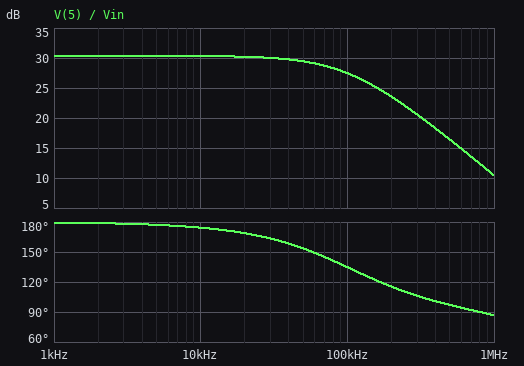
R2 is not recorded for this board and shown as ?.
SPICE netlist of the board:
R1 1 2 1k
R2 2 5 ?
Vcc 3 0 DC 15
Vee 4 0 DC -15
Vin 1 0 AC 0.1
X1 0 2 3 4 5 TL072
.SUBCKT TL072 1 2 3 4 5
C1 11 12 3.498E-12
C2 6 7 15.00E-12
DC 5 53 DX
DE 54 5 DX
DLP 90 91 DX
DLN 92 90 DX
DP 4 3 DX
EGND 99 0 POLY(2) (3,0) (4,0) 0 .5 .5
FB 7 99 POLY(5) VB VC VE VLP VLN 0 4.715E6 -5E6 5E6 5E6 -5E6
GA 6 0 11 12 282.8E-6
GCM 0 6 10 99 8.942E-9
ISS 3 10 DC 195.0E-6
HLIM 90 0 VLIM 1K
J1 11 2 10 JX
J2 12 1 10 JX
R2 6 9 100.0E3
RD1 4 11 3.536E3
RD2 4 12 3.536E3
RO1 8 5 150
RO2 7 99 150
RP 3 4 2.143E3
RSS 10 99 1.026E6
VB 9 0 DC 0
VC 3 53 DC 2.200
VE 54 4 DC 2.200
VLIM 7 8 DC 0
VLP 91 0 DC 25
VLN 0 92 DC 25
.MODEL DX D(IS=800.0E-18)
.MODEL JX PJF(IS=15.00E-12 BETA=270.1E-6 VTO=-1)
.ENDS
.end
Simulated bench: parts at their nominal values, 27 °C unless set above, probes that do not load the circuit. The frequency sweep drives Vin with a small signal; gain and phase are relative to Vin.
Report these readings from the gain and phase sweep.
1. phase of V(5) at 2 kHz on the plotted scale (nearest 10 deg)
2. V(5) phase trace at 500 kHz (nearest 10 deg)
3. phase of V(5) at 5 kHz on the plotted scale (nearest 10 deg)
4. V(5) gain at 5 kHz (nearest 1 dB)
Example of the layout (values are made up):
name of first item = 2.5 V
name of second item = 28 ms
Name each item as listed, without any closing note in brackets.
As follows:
phase of V(5) at 2 kHz on the plotted scale = 180 deg
V(5) phase trace at 500 kHz = 100 deg
phase of V(5) at 5 kHz on the plotted scale = 180 deg
V(5) gain at 5 kHz = 30 dB
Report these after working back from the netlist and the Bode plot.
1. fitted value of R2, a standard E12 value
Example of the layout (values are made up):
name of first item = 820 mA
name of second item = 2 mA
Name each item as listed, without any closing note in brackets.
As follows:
fitted value of R2, a standard E12 value = 33 kΩ
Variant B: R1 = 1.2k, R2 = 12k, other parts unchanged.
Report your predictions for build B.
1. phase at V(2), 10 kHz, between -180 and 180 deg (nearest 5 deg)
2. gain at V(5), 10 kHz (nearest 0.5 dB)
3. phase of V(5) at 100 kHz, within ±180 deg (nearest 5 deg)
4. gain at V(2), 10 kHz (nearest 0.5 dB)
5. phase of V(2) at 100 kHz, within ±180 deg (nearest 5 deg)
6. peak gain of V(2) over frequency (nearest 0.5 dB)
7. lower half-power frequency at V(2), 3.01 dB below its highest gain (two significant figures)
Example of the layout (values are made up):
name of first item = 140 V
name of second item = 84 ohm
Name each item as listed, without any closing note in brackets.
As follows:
phase at V(2), 10 kHz, between -180 and 180 deg = 90 deg
gain at V(5), 10 kHz = 20.0 dB
phase of V(5) at 100 kHz, within ±180 deg = 160 deg
gain at V(2), 10 kHz = -30.5 dB
phase of V(2) at 100 kHz, within ±180 deg = 75 deg
peak gain of V(2) over frequency = -0.5 dB
lower half-power frequency at V(2), 3.01 dB below its highest gain = 320 kHz
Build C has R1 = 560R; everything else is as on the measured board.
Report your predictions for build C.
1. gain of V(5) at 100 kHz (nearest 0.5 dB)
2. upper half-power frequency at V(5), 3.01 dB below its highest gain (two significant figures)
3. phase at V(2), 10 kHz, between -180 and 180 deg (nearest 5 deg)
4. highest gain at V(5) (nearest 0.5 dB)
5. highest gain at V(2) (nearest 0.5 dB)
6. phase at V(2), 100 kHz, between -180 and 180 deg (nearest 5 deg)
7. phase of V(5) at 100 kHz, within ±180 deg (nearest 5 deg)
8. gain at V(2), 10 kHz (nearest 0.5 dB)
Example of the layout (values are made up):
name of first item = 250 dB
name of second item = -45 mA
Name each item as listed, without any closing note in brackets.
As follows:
gain of V(5) at 100 kHz = 29.5 dB
upper half-power frequency at V(5), 3.01 dB below its highest gain = 58 kHz
phase at V(2), 10 kHz, between -180 and 180 deg = 80 deg
highest gain at V(5) = 35.5 dB
highest gain at V(2) = 0 dB
phase at V(2), 100 kHz, between -180 and 180 deg = 30 deg
phase of V(5) at 100 kHz, within ±180 deg = 120 deg
gain at V(2), 10 kHz = -15.5 dB
